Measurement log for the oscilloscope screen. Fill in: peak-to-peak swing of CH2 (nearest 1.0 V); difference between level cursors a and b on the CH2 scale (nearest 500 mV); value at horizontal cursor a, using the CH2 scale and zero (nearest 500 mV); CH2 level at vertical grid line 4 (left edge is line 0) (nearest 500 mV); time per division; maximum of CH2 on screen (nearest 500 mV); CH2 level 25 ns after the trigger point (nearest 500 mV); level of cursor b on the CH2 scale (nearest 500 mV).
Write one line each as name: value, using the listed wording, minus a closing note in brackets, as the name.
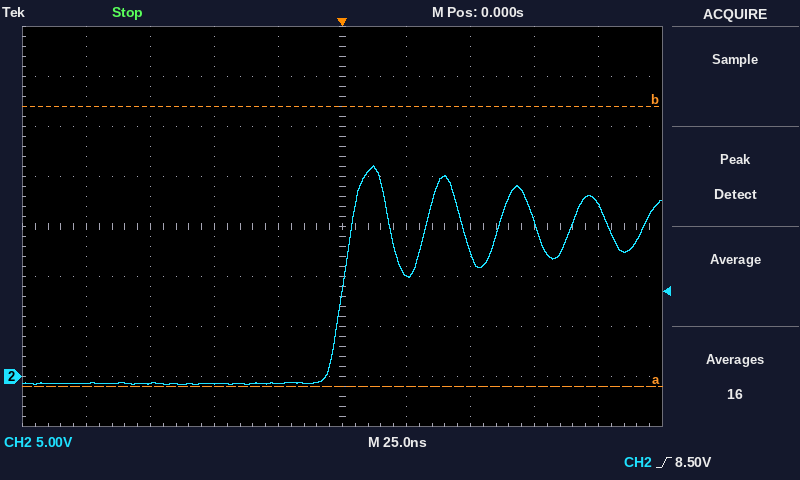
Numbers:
peak-to-peak swing of CH2: 22.0 V
difference between level cursors a and b on the CH2 scale: 28.0 V
value at horizontal cursor a, using the CH2 scale and zero: -1.0 V
CH2 level at vertical grid line 4 (left edge is line 0): -500 mV
time per division: 25 ns
maximum of CH2 on screen: 21.0 V
CH2 level 25 ns after the trigger point: 10.0 V
level of cursor b on the CH2 scale: 27.0 V
